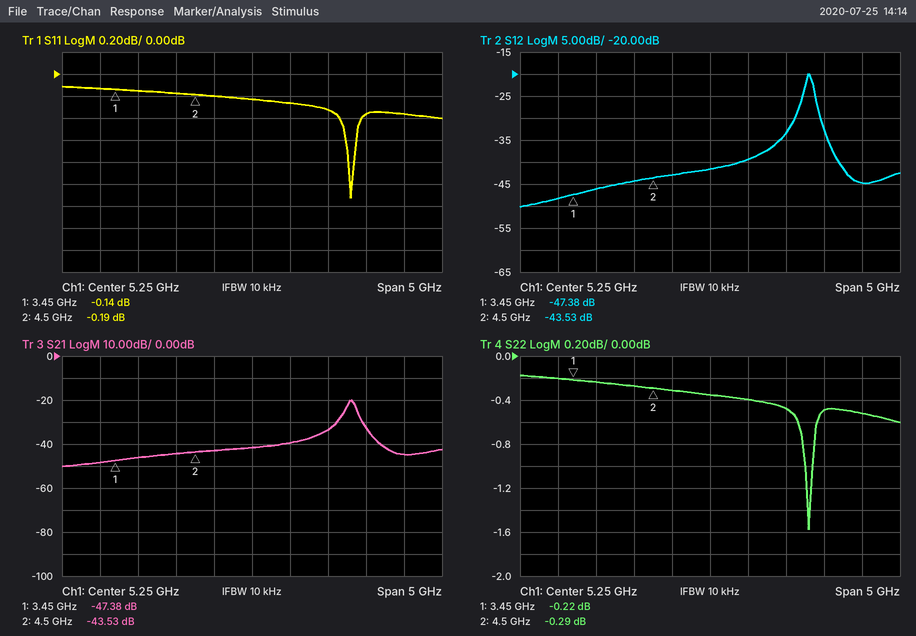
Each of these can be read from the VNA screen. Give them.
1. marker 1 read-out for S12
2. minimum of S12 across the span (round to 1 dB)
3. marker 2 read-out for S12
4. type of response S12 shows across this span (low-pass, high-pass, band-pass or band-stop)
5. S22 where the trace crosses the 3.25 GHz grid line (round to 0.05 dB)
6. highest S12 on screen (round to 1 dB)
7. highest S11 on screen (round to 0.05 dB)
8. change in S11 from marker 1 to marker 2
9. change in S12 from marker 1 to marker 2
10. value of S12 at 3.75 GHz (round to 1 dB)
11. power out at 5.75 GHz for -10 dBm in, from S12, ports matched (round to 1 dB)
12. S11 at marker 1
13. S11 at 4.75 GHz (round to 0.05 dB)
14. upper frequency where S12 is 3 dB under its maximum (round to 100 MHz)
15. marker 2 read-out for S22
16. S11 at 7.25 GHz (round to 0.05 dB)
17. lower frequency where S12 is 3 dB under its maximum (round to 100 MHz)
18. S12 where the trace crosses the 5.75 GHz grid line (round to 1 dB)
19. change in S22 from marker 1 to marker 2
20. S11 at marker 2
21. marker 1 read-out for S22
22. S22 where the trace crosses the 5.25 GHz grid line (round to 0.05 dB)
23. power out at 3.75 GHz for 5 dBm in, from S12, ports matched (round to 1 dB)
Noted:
-47.38 dB
-50 dB
-43.53 dB
band-pass
-0.20 dB
-20 dB
-0.10 dB
-0.05 dB
3.85 dB
-46 dB
-49 dBm
-0.14 dB
-0.20 dB
6.6 GHz
-0.29 dB
-0.35 dB
6.5 GHz
-39 dB
-0.07 dB
-0.19 dB
-0.22 dB
-0.35 dB
-41 dBm
